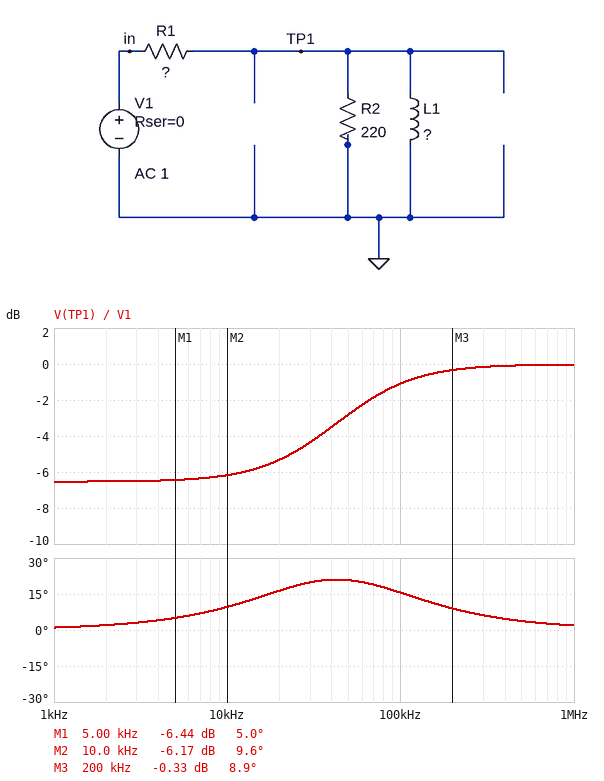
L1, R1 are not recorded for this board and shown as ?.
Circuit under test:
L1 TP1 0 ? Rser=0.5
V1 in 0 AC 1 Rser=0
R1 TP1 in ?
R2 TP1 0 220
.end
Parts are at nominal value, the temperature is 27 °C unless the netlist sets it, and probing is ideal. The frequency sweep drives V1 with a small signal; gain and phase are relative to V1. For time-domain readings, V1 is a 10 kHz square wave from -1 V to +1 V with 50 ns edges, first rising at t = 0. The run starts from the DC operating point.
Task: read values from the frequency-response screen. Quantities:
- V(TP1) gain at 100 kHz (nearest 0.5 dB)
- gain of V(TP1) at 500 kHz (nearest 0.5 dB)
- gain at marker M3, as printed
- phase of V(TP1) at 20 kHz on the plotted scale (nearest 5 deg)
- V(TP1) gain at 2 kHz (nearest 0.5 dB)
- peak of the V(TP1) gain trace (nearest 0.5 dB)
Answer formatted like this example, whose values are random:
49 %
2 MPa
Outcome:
-1.0 dB
0 dB
-0.33 dB
15 deg
-6.5 dB
0 dB
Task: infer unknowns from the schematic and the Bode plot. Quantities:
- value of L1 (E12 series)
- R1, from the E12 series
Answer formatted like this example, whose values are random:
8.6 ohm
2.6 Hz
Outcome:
2.7 µH
0.56 Ω
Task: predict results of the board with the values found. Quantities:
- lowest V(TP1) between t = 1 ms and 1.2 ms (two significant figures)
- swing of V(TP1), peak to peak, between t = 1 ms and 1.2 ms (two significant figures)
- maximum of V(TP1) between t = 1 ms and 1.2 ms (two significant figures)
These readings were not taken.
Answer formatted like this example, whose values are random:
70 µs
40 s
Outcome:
-1.5 V
3.0 V
1.5 V
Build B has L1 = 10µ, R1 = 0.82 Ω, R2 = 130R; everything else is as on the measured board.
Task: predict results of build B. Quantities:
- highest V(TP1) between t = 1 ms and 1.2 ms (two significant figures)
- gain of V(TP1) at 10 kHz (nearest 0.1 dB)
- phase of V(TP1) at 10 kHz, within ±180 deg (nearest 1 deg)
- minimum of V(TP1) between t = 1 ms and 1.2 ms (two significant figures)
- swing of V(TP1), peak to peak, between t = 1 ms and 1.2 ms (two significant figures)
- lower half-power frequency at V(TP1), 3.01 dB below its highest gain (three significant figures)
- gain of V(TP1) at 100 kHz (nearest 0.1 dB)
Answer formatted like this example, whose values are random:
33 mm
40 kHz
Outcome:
1.6 V
-5.2 dB
26 deg
-1.6 V
3.2 V
17.6 kHz
-0.2 dB
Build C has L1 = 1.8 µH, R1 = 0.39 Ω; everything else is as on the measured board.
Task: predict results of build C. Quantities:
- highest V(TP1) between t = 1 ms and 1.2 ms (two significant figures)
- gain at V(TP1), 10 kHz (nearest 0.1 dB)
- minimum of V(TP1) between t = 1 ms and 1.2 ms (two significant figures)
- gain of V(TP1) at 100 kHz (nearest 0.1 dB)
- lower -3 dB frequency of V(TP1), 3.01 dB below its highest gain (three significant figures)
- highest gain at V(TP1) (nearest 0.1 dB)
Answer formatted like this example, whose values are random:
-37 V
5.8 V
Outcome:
1.4 V
-4.9 dB
-1.4 V
-1.3 dB
47.7 kHz
0 dB
